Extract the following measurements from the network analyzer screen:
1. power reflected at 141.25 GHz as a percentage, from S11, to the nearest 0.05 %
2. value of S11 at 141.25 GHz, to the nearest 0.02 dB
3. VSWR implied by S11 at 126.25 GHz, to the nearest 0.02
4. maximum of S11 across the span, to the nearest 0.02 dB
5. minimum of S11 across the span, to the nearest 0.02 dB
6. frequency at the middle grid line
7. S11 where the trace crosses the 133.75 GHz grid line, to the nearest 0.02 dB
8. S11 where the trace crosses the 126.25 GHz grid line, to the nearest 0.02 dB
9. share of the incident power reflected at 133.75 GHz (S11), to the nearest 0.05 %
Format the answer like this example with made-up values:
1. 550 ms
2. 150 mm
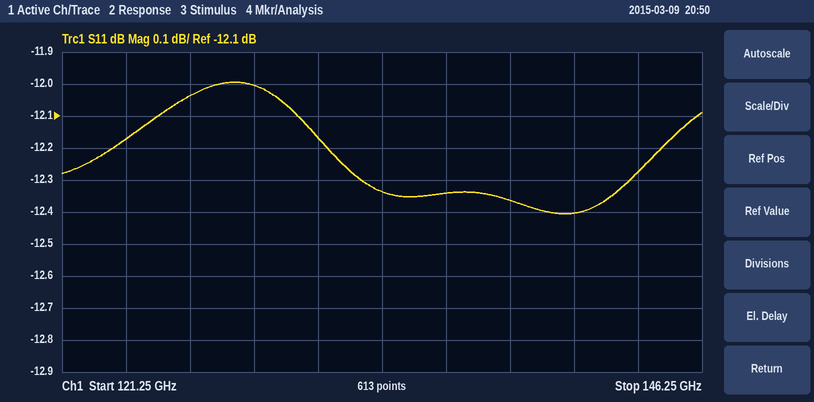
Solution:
1. 5.75 %
2. -12.40 dB
3. 1.66
4. -12.00 dB
5. -12.40 dB
6. 133.75 GHz
7. -12.34 dB
8. -12.04 dB
9. 5.85 %
